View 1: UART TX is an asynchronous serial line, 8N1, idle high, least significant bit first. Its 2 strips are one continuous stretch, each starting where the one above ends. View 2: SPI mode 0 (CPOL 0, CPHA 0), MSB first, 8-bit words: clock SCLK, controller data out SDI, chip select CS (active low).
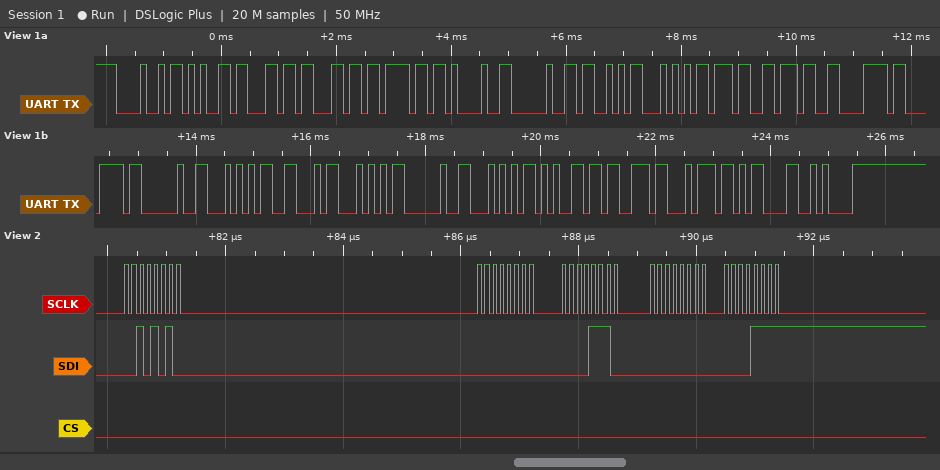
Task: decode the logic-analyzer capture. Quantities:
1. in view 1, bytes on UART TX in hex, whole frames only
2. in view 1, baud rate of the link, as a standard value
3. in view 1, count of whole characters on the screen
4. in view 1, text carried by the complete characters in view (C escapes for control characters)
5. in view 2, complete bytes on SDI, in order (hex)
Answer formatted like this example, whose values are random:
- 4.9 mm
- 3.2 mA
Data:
- 48 65 6C 6C 6F 21 20 53 54 37 37 78 78 20 54 46 54 20 54 65 73 74 0D 0A
- 9600 baud
- 24
- "Hello! ST77xx TFT Test\r\n"
- 2A 00 0E 00 0F
